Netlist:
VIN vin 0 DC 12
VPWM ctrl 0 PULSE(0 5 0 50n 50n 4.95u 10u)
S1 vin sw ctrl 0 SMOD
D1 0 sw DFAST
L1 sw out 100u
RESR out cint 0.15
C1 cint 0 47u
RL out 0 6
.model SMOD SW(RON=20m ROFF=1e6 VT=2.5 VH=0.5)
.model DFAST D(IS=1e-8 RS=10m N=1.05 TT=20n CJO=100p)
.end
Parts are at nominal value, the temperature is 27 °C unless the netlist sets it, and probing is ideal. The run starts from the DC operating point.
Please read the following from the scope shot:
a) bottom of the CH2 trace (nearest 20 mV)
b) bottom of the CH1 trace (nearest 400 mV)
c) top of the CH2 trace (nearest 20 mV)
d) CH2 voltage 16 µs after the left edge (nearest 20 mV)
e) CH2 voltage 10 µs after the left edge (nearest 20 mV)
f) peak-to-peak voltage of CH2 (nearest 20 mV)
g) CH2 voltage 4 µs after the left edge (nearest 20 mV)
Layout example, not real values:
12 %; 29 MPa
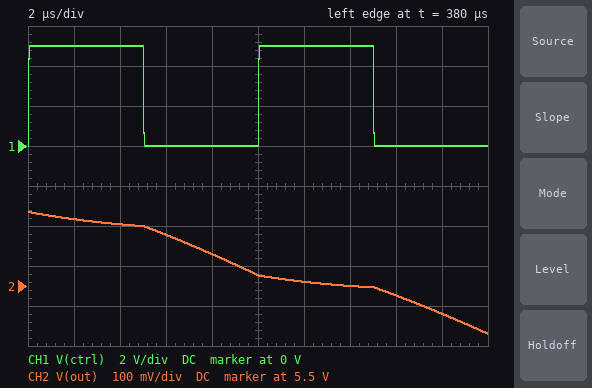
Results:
5.38 V; 0 V; 5.68 V; 5.48 V; 5.52 V; 300 mV; 5.66 V
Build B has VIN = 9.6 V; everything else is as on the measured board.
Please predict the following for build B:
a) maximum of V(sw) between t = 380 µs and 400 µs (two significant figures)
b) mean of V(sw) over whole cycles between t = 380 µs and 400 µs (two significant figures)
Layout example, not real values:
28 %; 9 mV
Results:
9.6 V; 4.6 V
